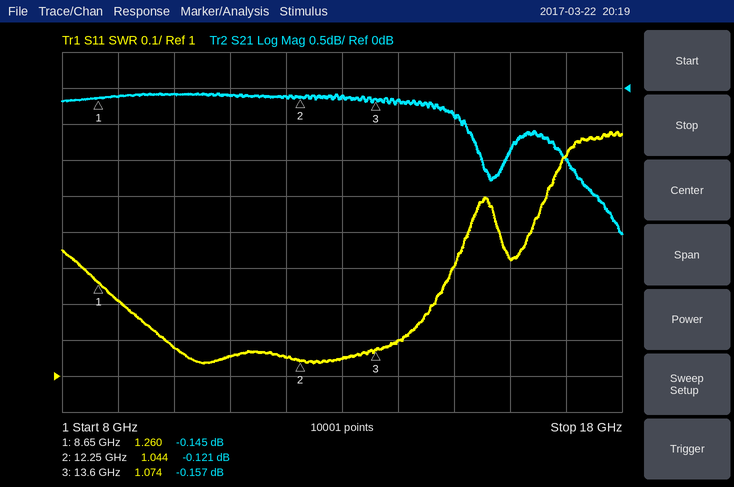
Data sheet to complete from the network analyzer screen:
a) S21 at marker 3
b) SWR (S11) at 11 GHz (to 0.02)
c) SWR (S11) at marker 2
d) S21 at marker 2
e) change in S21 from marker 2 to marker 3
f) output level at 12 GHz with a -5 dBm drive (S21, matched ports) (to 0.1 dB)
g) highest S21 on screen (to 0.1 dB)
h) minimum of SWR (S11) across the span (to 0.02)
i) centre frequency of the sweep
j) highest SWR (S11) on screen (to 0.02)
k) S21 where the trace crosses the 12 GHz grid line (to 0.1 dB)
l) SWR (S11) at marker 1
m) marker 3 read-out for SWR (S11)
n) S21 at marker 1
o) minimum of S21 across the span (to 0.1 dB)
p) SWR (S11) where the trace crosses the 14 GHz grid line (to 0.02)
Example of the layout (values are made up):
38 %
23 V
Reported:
-0.157 dB
1.06
1.044
-0.121 dB
-0.036 dB
-5.1 dBm
-0.1 dB
1.04
13 GHz
1.68
-0.1 dB
1.260
1.074
-0.145 dB
-2.0 dB
1.10
